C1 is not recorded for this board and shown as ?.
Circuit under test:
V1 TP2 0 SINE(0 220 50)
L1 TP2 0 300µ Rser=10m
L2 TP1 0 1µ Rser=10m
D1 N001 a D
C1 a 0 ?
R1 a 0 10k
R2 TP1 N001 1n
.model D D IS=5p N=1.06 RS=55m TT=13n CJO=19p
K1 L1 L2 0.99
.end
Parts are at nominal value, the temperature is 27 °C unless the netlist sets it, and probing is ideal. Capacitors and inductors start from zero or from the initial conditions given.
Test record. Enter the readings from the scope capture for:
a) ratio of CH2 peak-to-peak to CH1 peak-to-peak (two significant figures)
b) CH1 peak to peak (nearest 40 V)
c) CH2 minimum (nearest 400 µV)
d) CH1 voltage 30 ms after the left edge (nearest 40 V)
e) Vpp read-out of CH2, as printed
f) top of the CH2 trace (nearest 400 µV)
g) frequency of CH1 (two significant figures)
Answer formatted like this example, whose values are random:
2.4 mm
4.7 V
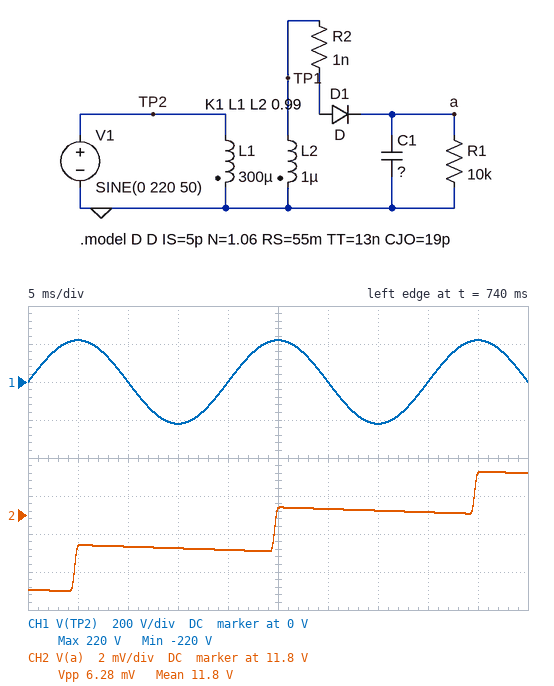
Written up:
0.000014
440 V
11.7940 V
0 V
6.28 mV
11.8004 V
50 Hz
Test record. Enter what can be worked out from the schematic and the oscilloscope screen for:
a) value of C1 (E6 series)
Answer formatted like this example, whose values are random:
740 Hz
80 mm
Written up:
68 mF
